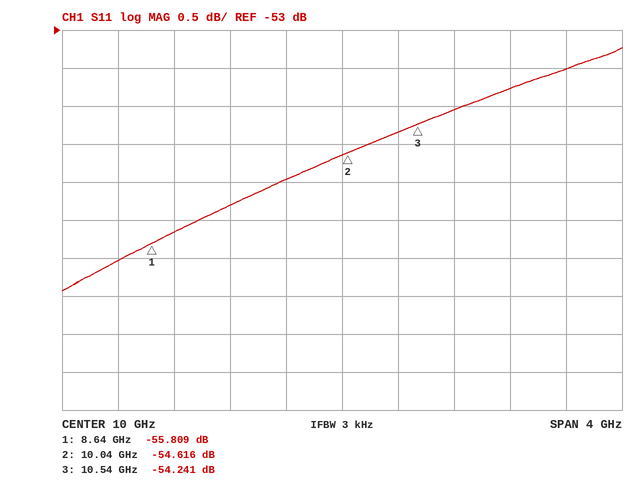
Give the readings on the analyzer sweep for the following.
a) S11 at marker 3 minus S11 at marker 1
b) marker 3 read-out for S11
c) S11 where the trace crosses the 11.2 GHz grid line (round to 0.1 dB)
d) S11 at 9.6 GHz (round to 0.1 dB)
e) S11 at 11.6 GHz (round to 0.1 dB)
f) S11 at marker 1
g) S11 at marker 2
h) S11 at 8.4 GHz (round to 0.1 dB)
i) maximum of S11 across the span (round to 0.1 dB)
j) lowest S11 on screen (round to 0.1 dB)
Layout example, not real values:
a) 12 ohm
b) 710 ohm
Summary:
a) 1.568 dB
b) -54.241 dB
c) -53.8 dB
d) -55.0 dB
e) -53.5 dB
f) -55.809 dB
g) -54.616 dB
h) -56.0 dB
i) -53.2 dB
j) -56.4 dB
